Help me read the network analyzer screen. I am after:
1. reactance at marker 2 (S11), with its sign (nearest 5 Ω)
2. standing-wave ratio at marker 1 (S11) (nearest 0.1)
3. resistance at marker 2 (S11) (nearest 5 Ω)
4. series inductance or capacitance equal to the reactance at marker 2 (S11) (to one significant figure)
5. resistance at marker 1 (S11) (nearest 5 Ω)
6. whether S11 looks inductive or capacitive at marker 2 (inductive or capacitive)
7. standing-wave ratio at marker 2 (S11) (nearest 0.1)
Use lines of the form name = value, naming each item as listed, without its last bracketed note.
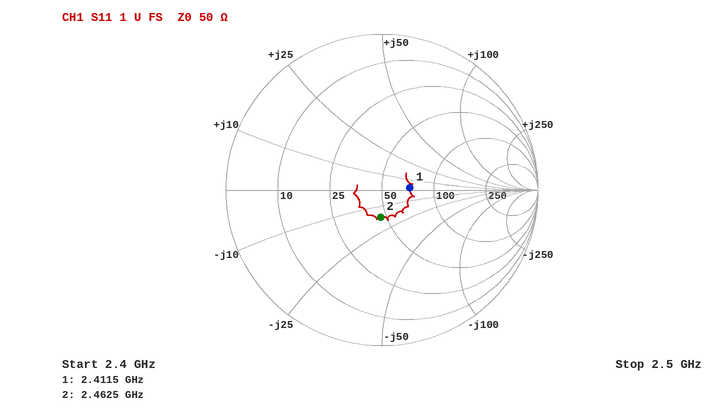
reactance at marker 2 (S11), with its sign = -15 Ω
standing-wave ratio at marker 1 (S11) = 1.4
resistance at marker 2 (S11) = 45 Ω
series inductance or capacitance equal to the reactance at marker 2 (S11) = 4 pF
resistance at marker 1 (S11) = 70 Ω
whether S11 looks inductive or capacitive at marker 2 = capacitive
standing-wave ratio at marker 2 (S11) = 1.4
